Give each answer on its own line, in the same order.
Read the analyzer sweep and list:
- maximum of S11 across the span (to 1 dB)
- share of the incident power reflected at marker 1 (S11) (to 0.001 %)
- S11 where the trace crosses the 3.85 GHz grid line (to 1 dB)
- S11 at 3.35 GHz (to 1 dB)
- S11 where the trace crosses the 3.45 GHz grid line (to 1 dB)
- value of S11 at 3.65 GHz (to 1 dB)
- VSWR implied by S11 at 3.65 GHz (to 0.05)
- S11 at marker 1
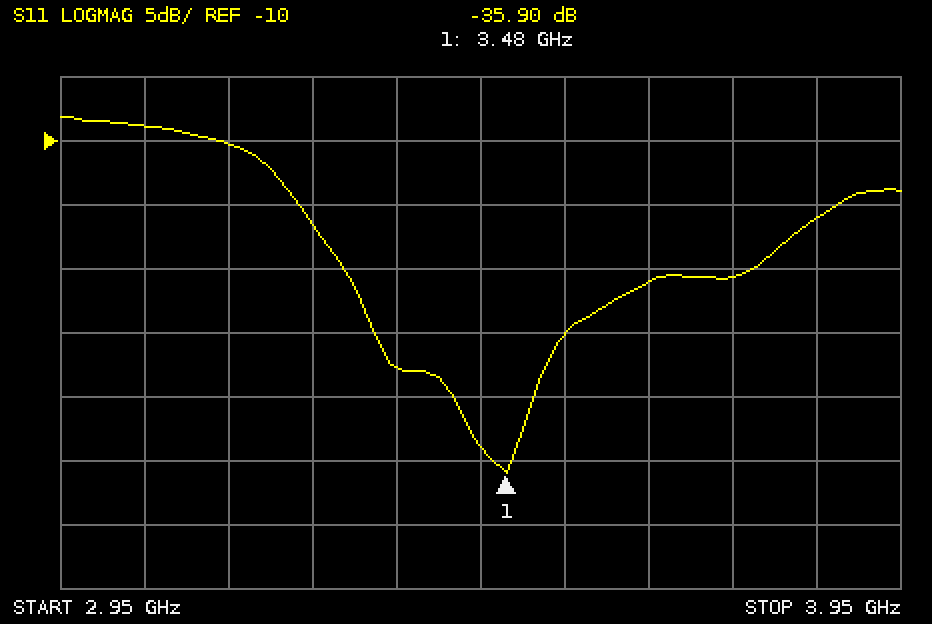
-8 dB
0.026 %
-16 dB
-28 dB
-34 dB
-21 dB
1.20
-35.90 dB
